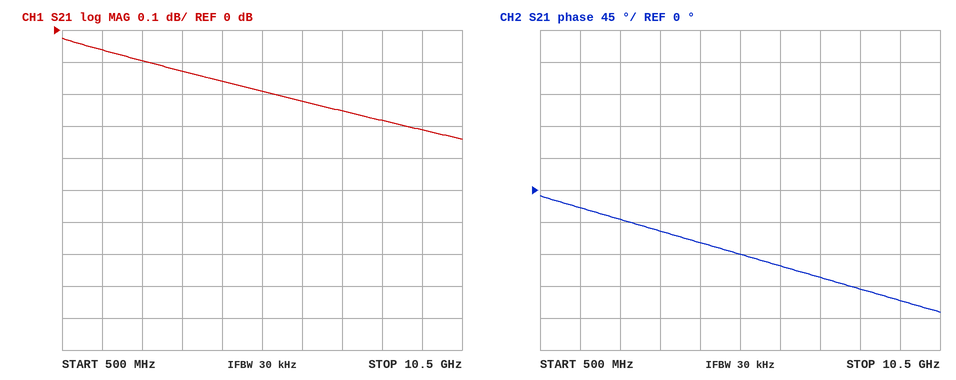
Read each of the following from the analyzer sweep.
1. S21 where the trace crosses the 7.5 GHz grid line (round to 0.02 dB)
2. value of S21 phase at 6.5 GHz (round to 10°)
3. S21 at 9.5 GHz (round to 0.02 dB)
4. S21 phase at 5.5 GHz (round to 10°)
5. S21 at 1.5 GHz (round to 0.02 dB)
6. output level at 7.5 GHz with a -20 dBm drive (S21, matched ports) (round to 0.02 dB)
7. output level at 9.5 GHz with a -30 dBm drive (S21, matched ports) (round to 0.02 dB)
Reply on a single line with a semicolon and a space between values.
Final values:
-0.26 dB; -110°; -0.32 dB; -90°; -0.06 dB; -20.26 dBm; -30.32 dBm
